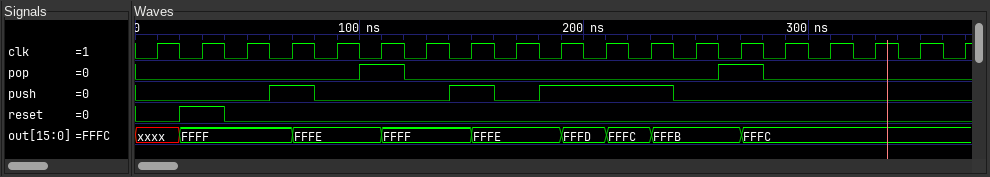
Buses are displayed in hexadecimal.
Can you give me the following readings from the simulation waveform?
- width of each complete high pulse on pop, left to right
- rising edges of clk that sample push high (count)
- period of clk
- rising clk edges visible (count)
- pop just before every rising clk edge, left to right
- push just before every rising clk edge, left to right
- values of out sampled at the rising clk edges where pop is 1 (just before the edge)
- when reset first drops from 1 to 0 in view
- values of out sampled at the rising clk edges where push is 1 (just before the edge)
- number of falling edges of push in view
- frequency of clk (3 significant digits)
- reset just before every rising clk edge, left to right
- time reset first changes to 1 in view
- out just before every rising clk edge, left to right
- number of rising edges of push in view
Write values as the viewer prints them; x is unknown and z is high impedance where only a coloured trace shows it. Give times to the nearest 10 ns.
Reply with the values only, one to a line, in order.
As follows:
20 ns, 20 ns
5
20 ns
19
0 0 0 0 0 1 0 0 0 0 0 0 0 1 0 0 0 0 0
0 0 0 1 0 0 0 1 0 1 1 1 0 0 0 0 0 0 0
FFFE, FFFB
40 ns
FFFF, FFFF, FFFE, FFFD, FFFC
3
50.0 MHz
0 1 0 0 0 0 0 0 0 0 0 0 0 0 0 0 0 0 0
20 ns
xxxx, FFFF, FFFF, FFFF, FFFE, FFFE, FFFF, FFFF, FFFE, FFFE, FFFD, FFFC, FFFB, FFFB, FFFC, FFFC, FFFC, FFFC, FFFC
3
